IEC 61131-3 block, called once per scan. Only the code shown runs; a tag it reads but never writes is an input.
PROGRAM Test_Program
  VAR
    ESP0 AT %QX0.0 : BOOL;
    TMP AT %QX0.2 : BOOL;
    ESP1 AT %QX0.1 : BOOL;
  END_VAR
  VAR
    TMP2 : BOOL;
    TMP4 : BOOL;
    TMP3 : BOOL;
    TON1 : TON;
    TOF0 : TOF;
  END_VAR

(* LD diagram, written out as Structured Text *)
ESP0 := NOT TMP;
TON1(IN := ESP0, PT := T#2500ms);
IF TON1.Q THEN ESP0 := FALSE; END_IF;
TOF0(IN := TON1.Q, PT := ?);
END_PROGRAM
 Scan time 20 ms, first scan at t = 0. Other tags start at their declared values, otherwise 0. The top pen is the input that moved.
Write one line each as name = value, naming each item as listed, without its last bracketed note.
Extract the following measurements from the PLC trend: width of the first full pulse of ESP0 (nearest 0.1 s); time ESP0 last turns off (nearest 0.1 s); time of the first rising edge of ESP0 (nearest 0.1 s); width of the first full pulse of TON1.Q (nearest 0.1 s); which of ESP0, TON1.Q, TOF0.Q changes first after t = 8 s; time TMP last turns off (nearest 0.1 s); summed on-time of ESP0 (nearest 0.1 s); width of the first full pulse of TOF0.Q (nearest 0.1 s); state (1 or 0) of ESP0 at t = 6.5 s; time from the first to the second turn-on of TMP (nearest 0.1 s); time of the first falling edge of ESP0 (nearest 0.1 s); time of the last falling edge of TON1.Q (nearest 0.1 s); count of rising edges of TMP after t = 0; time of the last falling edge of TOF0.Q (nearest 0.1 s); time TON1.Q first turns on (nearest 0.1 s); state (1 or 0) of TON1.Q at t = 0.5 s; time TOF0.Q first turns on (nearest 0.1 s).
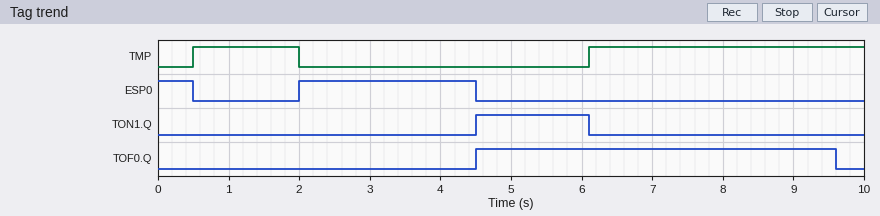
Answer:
width of the first full pulse of ESP0 = 2.5 s
time ESP0 last turns off = 4.5 s
time of the first rising edge of ESP0 = 2.0 s
width of the first full pulse of TON1.Q = 1.6 s
which of ESP0, TON1.Q, TOF0.Q changes first after t = 8 s = TOF0.Q
time TMP last turns off = 2.0 s
summed on-time of ESP0 = 3.0 s
width of the first full pulse of TOF0.Q = 5.1 s
state (1 or 0) of ESP0 at t = 6.5 s = 0
time from the first to the second turn-on of TMP = 5.6 s
time of the first falling edge of ESP0 = 0.5 s
time of the last falling edge of TON1.Q = 6.1 s
count of rising edges of TMP after t = 0 = 2
time of the last falling edge of TOF0.Q = 9.6 s
time TON1.Q first turns on = 4.5 s
state (1 or 0) of TON1.Q at t = 0.5 s = 0
time TOF0.Q first turns on = 4.5 s
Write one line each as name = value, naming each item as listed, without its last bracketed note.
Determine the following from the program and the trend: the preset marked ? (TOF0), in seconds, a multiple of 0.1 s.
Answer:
the preset marked ? (TOF0), in seconds, a multiple of 0.1 s = 3.5 s
